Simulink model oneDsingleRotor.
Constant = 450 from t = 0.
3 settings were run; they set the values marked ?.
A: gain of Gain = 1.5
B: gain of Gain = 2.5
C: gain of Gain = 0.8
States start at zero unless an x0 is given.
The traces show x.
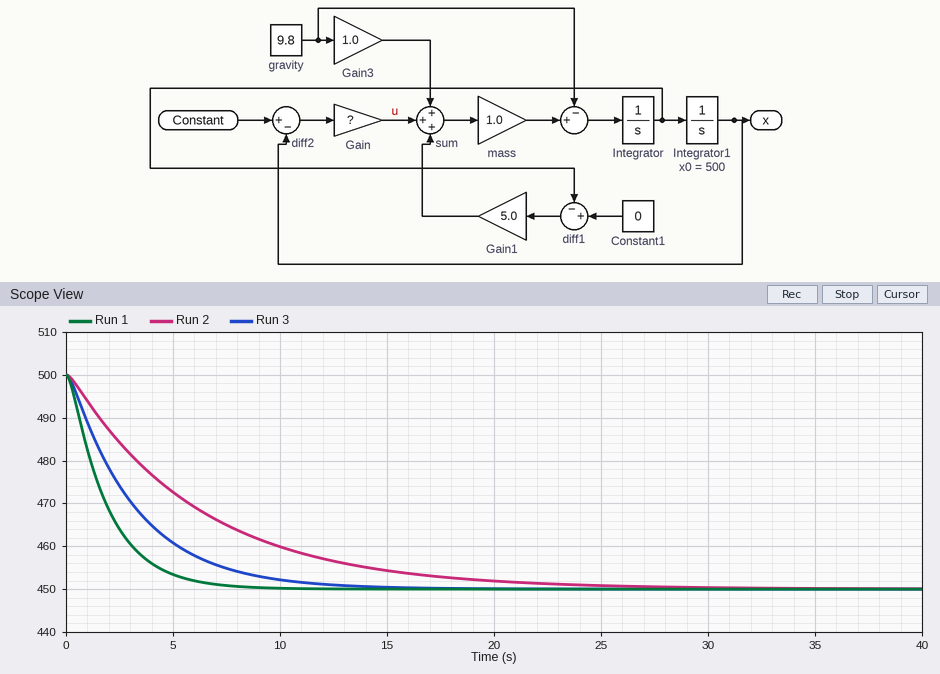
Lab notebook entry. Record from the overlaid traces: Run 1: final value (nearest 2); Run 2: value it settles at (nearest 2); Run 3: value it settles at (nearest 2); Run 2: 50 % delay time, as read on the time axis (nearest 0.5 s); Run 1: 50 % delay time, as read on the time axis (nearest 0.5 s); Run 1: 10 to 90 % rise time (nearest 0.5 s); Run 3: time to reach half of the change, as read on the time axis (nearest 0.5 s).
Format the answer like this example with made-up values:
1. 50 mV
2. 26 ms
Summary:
1. 450
2. 450
3. 450
4. 4.5 s
5. 1.5 s
6. 4.0 s
7. 2.5 s
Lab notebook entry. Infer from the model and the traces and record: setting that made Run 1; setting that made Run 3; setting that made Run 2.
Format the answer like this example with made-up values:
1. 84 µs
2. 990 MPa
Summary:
1. B
2. A
3. C
